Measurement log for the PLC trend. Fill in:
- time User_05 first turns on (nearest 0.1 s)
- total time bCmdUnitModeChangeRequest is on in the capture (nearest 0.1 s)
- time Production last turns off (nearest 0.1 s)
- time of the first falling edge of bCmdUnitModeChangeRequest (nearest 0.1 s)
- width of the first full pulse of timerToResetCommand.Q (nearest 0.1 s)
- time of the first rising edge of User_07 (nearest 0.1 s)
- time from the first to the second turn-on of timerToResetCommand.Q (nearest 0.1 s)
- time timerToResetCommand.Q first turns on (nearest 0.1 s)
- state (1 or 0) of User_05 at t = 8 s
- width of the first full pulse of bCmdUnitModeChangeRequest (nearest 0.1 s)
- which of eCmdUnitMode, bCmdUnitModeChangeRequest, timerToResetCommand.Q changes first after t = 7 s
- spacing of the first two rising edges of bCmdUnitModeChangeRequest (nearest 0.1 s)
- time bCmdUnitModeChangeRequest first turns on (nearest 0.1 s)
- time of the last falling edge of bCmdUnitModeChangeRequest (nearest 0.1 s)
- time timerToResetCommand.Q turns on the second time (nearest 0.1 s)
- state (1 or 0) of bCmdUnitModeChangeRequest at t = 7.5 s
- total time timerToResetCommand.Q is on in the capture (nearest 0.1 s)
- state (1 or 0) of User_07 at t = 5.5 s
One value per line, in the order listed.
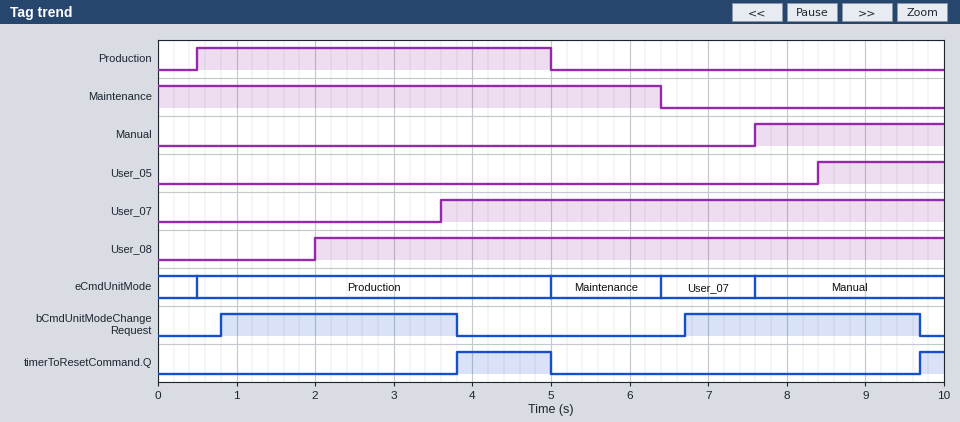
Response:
8.4 s
6.0 s
5.0 s
3.8 s
1.2 s
3.6 s
5.9 s
3.8 s
0
3.0 s
eCmdUnitMode
5.9 s
0.8 s
9.7 s
9.7 s
1
1.5 s
1
